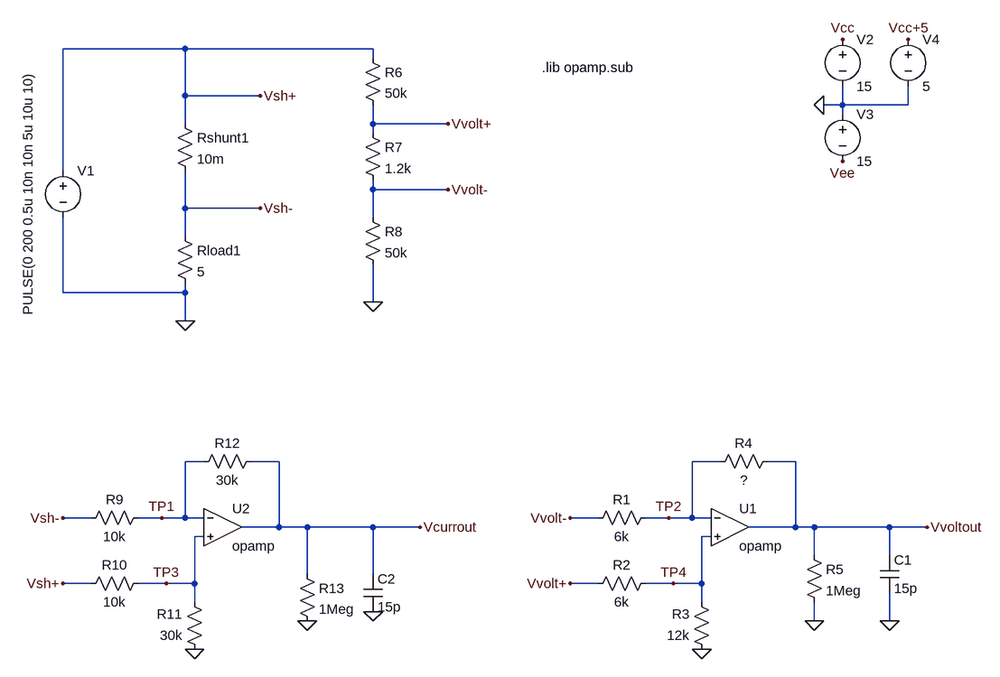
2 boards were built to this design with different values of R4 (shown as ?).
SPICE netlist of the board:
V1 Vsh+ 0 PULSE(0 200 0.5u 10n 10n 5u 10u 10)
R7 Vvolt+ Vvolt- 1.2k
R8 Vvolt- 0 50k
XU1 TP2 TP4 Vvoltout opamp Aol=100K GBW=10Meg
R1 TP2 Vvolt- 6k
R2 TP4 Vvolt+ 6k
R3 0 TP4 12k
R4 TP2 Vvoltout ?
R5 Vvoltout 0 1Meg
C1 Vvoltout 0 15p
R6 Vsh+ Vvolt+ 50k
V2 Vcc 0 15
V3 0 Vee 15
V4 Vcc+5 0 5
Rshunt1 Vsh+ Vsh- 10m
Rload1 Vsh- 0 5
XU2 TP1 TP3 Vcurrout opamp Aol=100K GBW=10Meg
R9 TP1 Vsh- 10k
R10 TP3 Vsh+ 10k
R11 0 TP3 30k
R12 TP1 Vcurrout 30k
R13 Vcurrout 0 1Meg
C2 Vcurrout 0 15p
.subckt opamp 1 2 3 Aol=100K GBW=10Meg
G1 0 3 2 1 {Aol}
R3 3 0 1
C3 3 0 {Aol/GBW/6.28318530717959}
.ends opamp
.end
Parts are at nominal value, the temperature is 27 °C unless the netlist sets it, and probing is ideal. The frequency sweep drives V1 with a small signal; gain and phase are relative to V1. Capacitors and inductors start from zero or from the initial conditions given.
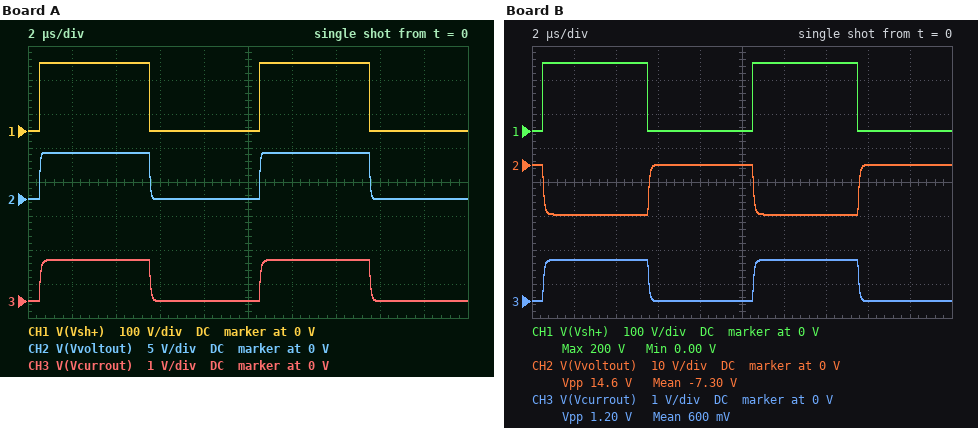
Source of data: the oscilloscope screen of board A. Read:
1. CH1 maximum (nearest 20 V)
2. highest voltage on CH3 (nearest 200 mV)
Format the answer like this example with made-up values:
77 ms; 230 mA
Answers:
200 V; 1.2 V
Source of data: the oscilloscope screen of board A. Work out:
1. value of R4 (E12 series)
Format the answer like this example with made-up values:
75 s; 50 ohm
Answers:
10 kΩ
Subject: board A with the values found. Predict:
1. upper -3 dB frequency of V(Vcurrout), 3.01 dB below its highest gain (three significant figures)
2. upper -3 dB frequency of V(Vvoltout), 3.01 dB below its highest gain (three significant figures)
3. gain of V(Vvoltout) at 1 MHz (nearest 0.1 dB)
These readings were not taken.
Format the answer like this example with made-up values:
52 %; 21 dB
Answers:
2.50 MHz; 3.81 MHz; -29.6 dB
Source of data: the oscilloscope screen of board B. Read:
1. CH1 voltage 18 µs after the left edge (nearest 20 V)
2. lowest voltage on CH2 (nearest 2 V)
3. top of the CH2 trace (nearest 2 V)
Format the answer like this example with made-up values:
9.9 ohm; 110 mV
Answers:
0 V; -14 V; 0 V
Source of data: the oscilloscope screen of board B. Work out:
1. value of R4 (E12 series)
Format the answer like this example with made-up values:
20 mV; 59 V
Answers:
27 kΩ
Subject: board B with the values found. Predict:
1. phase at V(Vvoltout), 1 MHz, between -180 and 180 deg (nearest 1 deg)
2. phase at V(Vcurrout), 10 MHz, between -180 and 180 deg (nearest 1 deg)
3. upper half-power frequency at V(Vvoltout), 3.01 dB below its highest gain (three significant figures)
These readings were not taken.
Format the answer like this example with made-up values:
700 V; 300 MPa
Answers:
157 deg; -76 deg; 2.34 MHz
